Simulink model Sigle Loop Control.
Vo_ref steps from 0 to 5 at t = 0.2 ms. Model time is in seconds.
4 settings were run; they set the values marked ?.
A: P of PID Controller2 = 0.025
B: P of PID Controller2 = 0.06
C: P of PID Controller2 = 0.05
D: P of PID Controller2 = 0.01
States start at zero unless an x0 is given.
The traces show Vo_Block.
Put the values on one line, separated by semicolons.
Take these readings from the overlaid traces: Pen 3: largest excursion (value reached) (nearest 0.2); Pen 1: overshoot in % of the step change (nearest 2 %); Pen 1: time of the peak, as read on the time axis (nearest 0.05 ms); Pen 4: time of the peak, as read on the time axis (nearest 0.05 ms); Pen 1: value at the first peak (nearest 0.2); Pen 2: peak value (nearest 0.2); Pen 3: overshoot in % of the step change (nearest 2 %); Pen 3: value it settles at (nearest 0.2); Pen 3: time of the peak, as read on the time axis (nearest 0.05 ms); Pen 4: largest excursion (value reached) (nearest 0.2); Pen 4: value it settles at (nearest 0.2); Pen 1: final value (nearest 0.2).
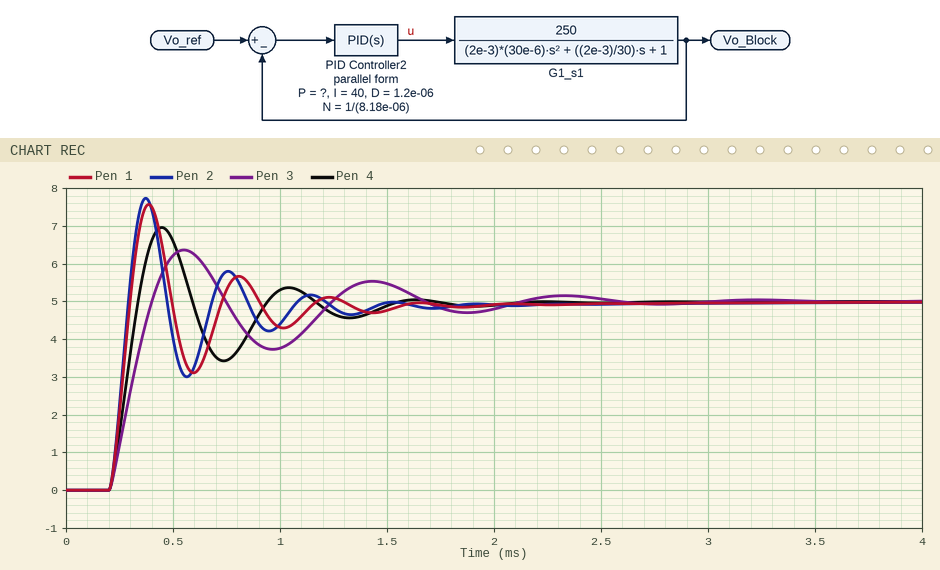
6.4; 52 %; 0.40 ms; 0.45 ms; 7.6; 7.8; 28 %; 5.0; 0.55 ms; 7.0; 5.0; 5.0
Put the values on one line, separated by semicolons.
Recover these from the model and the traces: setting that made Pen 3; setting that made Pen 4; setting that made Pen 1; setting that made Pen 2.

D; A; C; B
